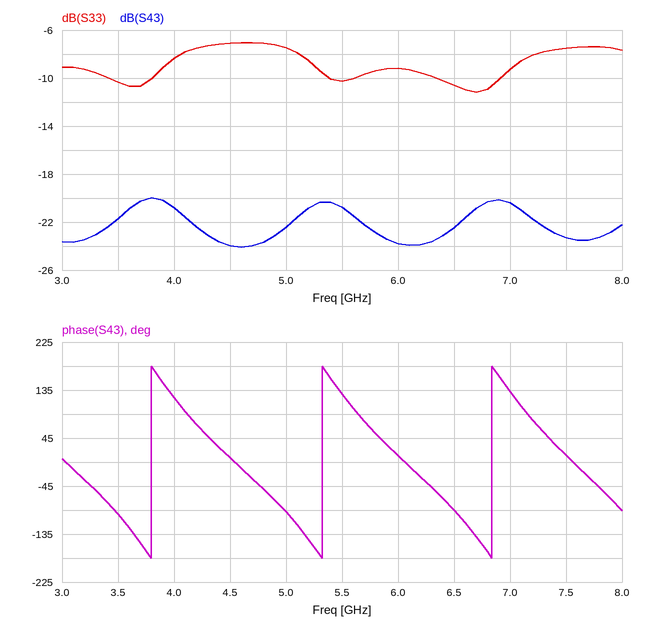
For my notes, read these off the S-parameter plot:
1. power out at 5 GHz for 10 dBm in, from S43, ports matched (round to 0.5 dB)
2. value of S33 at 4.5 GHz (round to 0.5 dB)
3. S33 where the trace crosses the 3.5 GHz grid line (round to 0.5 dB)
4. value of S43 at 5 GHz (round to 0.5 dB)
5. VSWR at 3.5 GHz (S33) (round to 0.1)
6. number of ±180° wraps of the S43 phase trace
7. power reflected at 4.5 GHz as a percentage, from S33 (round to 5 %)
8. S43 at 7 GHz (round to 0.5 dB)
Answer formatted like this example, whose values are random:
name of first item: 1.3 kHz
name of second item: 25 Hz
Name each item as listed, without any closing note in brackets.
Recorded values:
power out at 5 GHz for 10 dBm in, from S43, ports matched: -12.5 dBm
value of S33 at 4.5 GHz: -7.0 dB
S33 where the trace crosses the 3.5 GHz grid line: -10.5 dB
value of S43 at 5 GHz: -22.5 dB
VSWR at 3.5 GHz (S33): 1.9
number of ±180° wraps of the S43 phase trace: 3
power reflected at 4.5 GHz as a percentage, from S33: 20 %
S43 at 7 GHz: -20.5 dB
